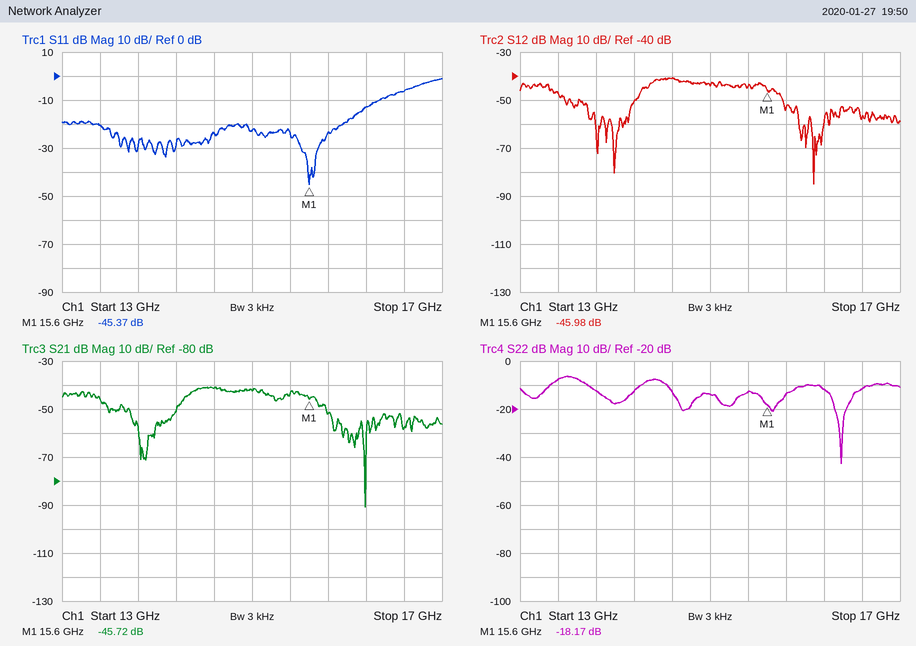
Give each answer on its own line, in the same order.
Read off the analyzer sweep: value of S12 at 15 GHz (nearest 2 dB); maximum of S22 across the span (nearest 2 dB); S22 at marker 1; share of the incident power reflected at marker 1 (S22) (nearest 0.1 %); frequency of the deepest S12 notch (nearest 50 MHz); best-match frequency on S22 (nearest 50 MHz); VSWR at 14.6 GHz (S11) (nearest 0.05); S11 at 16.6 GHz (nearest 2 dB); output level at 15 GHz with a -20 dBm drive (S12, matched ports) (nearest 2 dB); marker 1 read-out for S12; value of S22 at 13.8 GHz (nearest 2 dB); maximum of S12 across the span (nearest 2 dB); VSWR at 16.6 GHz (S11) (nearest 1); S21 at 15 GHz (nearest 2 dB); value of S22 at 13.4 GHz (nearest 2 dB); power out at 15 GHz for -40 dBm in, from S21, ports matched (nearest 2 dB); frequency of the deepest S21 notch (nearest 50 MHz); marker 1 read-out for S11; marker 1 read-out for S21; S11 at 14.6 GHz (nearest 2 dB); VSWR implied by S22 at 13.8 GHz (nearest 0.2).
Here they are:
-44 dB
-6 dB
-18.17 dB
1.5 %
16.10 GHz
16.40 GHz
1.15
-6 dB
-64 dBm
-45.98 dB
-12 dB
-40 dB
3
-42 dB
-8 dB
-82 dBm
16.20 GHz
-45.37 dB
-45.72 dB
-24 dB
1.6
